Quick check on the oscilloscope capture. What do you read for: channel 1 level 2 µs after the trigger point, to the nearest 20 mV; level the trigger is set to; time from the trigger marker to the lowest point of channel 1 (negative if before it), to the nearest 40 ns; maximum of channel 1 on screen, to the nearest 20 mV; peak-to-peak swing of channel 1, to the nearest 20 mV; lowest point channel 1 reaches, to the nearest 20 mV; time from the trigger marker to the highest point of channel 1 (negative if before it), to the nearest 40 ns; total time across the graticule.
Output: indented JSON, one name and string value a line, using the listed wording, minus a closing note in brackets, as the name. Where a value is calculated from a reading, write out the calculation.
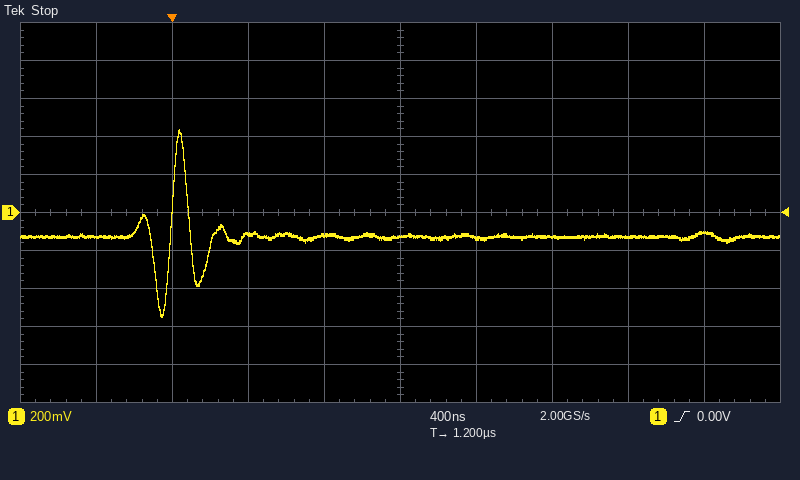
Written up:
{
  "channel 1 level 2 µs after the trigger point, to the nearest 20 mV": "-120 mV",
  "level the trigger is set to": "0.00 V",
  "time from the trigger marker to the lowest point of channel 1 (negative if before it), to the nearest 40 ns": "-40 ns",
  "maximum of channel 1 on screen, to the nearest 20 mV": "440 mV",
  "peak-to-peak swing of channel 1, to the nearest 20 mV": "440 mV − (-540 mV) = 980 mV",
  "lowest point channel 1 reaches, to the nearest 20 mV": "-540 mV",
  "time from the trigger marker to the highest point of channel 1 (negative if before it), to the nearest 40 ns": "+40 ns",
  "total time across the graticule": "4 µs"
}
